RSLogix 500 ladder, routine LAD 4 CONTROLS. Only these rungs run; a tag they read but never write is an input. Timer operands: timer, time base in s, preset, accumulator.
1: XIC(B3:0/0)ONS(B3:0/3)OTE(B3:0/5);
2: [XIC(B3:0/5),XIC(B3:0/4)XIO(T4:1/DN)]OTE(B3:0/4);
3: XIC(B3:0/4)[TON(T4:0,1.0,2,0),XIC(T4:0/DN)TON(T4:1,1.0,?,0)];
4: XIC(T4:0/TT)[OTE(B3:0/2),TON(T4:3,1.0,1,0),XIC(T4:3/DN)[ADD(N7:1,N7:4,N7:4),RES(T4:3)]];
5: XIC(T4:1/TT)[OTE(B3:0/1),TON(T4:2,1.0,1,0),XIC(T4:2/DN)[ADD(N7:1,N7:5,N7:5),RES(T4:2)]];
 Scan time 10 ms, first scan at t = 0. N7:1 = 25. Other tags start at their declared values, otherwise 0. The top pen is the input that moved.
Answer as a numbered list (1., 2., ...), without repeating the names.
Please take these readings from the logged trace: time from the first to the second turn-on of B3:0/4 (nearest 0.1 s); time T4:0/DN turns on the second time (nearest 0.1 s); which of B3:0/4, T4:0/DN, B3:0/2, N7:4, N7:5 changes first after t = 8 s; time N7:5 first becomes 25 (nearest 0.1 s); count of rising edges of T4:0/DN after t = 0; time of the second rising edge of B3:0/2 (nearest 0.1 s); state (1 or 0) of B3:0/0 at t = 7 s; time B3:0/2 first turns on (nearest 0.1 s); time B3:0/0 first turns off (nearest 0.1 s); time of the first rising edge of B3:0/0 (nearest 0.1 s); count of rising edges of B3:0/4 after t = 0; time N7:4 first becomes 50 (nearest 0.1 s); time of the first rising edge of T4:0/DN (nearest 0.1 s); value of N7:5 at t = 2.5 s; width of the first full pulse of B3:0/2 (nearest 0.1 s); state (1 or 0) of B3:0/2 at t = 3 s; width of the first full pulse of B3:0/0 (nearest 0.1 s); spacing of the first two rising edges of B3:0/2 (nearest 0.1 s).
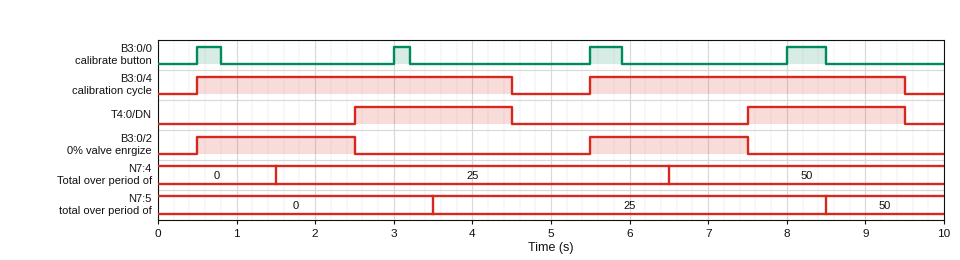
1. 5.0 s
2. 7.5 s
3. N7:5
4. 3.5 s
5. 2
6. 5.5 s
7. 0
8. 0.5 s
9. 0.8 s
10. 0.5 s
11. 2
12. 6.5 s
13. 2.5 s
14. 0
15. 2.0 s
16. 0
17. 0.3 s
18. 5.0 s
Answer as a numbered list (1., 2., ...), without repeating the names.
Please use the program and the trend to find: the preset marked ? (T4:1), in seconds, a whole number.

1. 2 s
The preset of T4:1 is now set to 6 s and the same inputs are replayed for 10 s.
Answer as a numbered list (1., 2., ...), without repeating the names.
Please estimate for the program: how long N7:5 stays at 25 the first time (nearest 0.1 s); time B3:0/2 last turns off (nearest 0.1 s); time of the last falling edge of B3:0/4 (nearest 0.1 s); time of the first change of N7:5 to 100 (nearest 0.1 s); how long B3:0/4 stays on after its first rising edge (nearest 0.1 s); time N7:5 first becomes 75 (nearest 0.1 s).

1. 1.0 s
2. 2.5 s
3. 8.5 s
4. 6.5 s
5. 8.0 s
6. 5.5 s
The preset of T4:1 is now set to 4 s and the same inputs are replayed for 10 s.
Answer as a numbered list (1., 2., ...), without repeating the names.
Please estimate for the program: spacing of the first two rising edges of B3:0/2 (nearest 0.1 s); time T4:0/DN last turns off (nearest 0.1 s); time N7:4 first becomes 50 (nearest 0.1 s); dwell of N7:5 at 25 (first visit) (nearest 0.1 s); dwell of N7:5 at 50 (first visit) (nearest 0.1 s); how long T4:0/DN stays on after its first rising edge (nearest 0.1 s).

1. 7.5 s
2. 6.5 s
3. 9.0 s
4. 1.0 s
5. 1.0 s
6. 4.0 s
